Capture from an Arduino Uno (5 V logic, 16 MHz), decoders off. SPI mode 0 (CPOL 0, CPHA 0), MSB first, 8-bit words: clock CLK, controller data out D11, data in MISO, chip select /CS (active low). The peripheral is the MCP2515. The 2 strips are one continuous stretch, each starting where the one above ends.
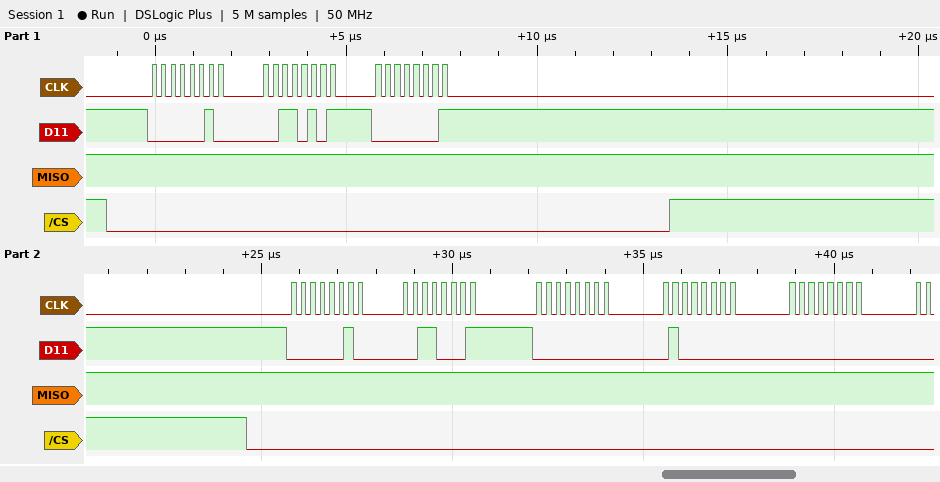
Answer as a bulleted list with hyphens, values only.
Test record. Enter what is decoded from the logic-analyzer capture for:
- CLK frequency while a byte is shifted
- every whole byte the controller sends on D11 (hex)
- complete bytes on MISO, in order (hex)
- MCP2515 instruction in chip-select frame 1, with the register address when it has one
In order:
- 4 MHz
- 02 35 01 02 31 00 40 00
- FF FF FF FF FF FF FF FF
- WRITE 0x35
